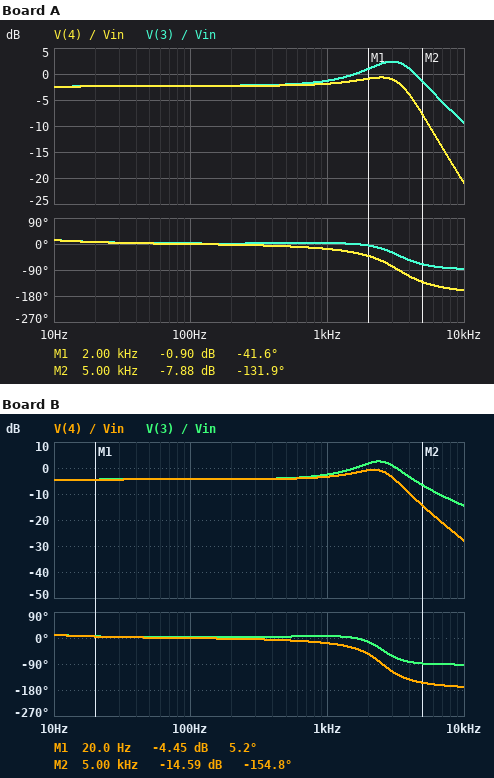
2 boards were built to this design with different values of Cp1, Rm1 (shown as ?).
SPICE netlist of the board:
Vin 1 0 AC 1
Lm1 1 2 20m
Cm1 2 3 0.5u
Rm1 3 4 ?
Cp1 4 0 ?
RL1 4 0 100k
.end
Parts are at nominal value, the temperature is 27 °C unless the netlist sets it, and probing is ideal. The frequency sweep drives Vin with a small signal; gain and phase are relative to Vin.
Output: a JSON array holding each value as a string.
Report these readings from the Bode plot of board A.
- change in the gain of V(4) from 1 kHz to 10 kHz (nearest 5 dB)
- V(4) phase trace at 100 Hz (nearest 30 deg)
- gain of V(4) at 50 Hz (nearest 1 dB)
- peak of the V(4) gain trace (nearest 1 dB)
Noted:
["-20 dB", "0 deg", "-2 dB", "-1 dB"]
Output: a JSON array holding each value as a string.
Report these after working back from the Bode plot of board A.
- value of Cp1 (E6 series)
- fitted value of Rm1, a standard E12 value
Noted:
["150 nF", "390 Ω"]
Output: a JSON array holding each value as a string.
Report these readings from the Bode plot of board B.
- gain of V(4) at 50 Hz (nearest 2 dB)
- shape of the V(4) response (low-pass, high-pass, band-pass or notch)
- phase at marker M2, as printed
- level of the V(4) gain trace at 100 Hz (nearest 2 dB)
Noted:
["-4 dB", "low-pass", "-154.8 deg", "-4 dB"]
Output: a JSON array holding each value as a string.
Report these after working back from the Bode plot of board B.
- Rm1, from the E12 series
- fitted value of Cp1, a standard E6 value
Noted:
["220 Ω", "330 nF"]
